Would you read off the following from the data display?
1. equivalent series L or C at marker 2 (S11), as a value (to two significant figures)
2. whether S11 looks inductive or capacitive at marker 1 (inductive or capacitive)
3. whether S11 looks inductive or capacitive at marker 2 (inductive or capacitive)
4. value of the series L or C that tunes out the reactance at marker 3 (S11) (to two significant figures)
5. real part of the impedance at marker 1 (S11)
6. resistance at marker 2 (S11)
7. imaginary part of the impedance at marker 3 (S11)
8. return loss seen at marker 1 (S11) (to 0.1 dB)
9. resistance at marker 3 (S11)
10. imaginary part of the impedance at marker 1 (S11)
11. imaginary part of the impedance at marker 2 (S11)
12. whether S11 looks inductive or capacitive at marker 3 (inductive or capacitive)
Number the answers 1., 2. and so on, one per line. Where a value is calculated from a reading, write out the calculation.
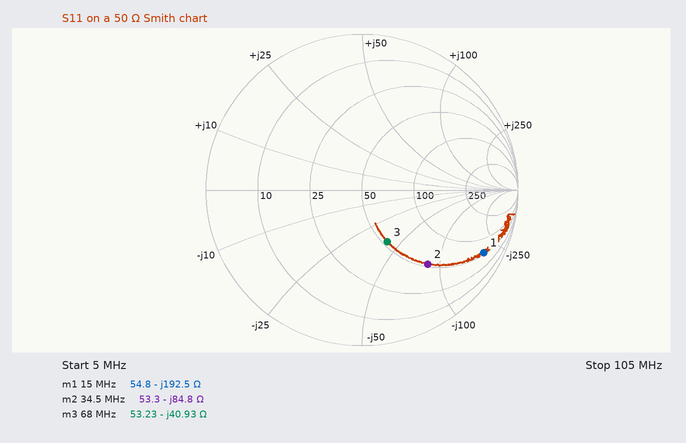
1. C = 1/(2π × 34.5 MHz × 84.8 Ω) ≈ 54 pF
2. capacitive
3. capacitive
4. L = 40.93 Ω/(2π × 68 MHz) ≈ 96 nH
5. 54.8 Ω
6. 53.3 Ω
7. -40.93 Ω
8. 1.1 dB
9. 53.23 Ω
10. -192.5 Ω
11. -84.8 Ω
12. capacitive
